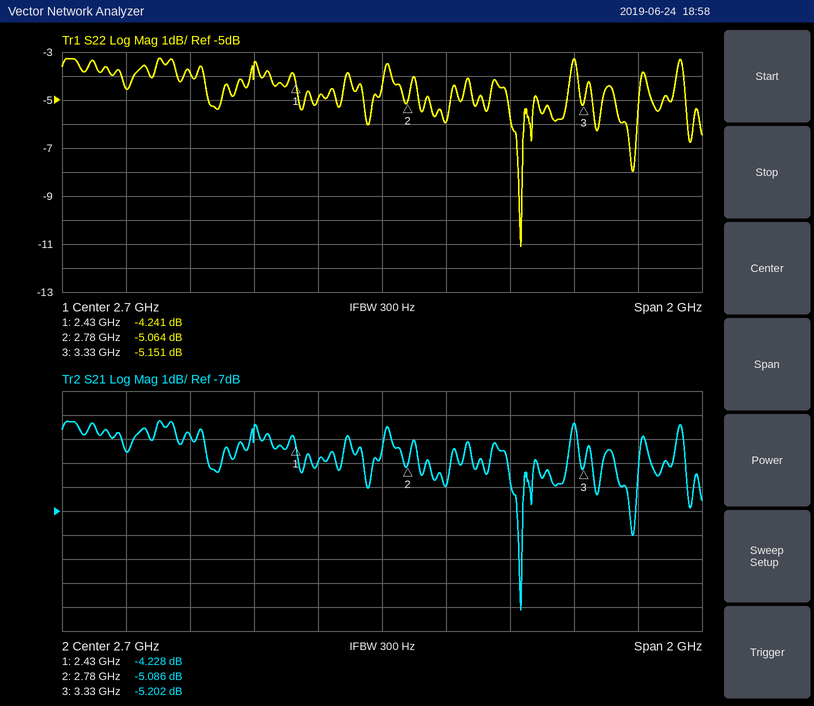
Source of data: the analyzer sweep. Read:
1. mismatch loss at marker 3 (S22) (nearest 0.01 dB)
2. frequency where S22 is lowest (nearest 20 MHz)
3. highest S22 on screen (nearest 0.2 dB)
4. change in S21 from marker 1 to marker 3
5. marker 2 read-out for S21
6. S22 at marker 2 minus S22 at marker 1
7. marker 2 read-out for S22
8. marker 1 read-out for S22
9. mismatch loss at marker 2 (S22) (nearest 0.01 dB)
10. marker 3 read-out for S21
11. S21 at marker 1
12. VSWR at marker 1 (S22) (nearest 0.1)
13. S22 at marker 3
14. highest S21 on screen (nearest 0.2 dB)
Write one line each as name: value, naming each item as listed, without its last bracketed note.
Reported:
mismatch loss at marker 3 (S22): 1.58 dB
frequency where S22 is lowest: 3.14 GHz
highest S22 on screen: -3.2 dB
change in S21 from marker 1 to marker 3: -0.974 dB
marker 2 read-out for S21: -5.086 dB
S22 at marker 2 minus S22 at marker 1: -0.823 dB
marker 2 read-out for S22: -5.064 dB
marker 1 read-out for S22: -4.241 dB
mismatch loss at marker 2 (S22): 1.62 dB
marker 3 read-out for S21: -5.202 dB
S21 at marker 1: -4.228 dB
VSWR at marker 1 (S22): 4.2
S22 at marker 3: -5.151 dB
highest S21 on screen: -3.2 dB
